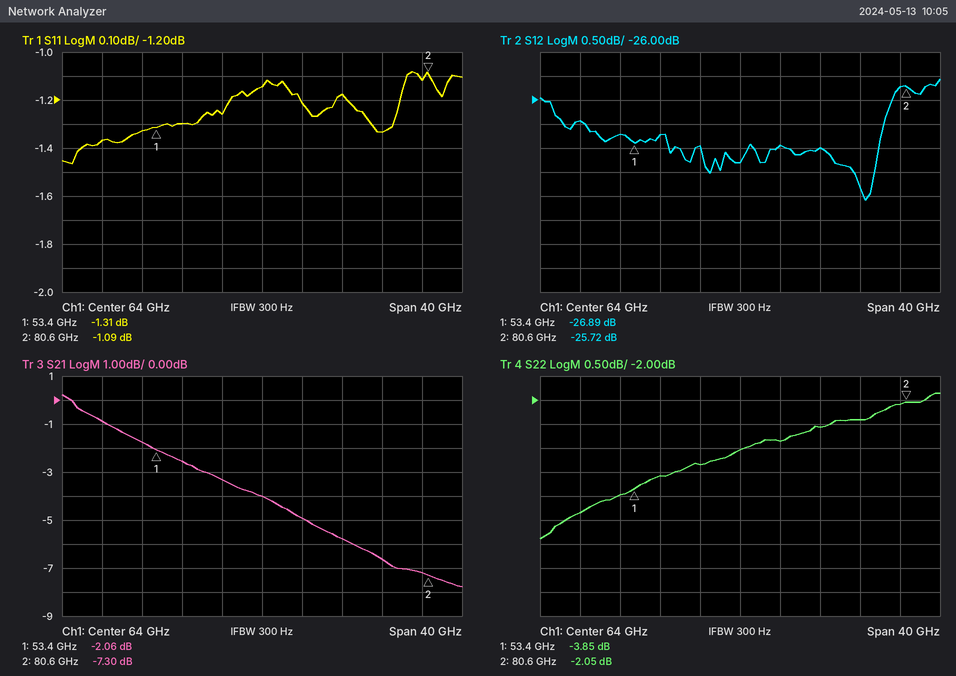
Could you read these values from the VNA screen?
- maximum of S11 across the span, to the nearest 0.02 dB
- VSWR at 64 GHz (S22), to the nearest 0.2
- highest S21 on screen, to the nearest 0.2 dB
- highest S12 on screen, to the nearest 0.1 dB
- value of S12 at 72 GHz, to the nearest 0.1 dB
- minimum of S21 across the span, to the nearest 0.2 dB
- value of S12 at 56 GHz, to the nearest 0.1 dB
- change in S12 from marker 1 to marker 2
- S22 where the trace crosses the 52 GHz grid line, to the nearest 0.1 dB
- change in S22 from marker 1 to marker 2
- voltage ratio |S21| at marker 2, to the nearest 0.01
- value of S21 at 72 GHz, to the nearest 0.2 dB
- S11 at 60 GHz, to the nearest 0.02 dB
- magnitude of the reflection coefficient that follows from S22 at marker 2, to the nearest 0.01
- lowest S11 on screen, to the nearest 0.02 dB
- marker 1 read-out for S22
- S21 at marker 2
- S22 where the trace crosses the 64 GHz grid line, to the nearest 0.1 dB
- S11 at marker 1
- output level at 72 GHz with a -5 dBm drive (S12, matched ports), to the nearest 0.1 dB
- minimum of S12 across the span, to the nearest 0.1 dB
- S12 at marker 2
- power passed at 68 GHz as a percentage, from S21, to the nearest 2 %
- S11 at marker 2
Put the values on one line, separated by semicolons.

-1.08 dB; 5.8; 0.2 dB; -25.6 dB; -27.0 dB; -7.8 dB; -26.7 dB; 1.17 dB; -4.0 dB; 1.80 dB; 0.43; -5.8 dB; -1.26 dB; 0.79; -1.46 dB; -3.85 dB; -7.30 dB; -3.0 dB; -1.31 dB; -32.0 dBm; -28.1 dB; -25.72 dB; 32 %; -1.09 dB
